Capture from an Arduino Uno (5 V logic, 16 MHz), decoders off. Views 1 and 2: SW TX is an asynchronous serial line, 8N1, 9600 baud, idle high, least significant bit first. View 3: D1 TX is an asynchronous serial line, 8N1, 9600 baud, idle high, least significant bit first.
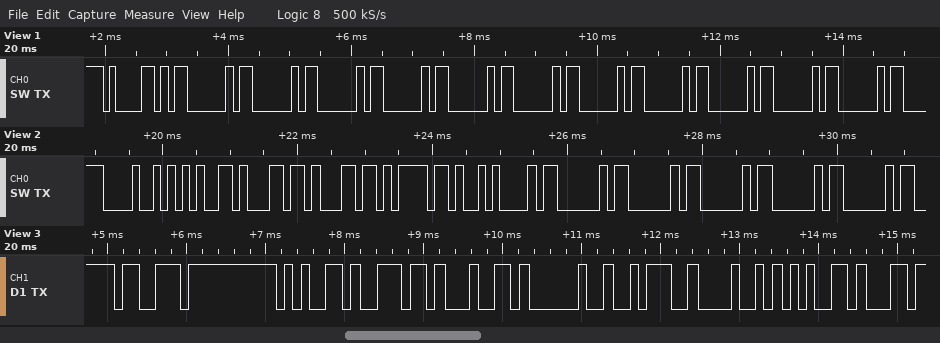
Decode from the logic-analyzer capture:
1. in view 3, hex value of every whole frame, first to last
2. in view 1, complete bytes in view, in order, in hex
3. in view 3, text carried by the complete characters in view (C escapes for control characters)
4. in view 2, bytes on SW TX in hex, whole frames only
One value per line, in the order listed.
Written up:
0x73 0x65 0x6E 0x64 0x20 0x3A 0x48 0x65
0x61 0x03 0x03 0x03 0x03 0x03 0x03 0x03 0x03 0x03 0x03 0x03
"send :He"
48 65 6C 6C 6F 0A 03 03 03 03 03
